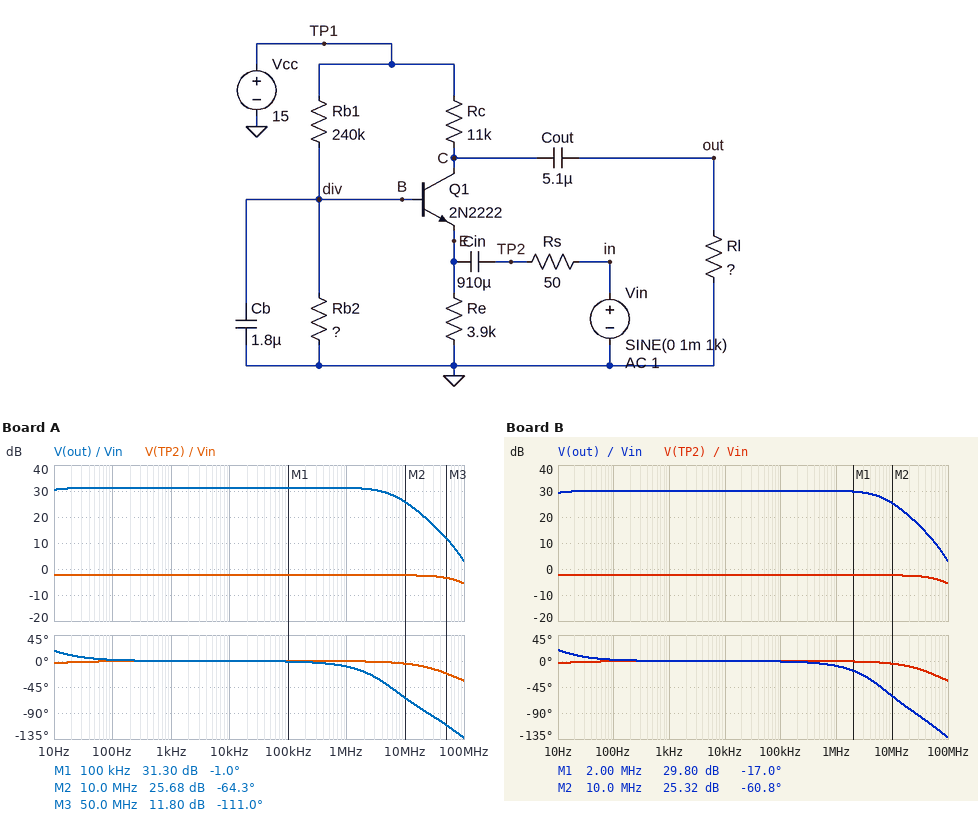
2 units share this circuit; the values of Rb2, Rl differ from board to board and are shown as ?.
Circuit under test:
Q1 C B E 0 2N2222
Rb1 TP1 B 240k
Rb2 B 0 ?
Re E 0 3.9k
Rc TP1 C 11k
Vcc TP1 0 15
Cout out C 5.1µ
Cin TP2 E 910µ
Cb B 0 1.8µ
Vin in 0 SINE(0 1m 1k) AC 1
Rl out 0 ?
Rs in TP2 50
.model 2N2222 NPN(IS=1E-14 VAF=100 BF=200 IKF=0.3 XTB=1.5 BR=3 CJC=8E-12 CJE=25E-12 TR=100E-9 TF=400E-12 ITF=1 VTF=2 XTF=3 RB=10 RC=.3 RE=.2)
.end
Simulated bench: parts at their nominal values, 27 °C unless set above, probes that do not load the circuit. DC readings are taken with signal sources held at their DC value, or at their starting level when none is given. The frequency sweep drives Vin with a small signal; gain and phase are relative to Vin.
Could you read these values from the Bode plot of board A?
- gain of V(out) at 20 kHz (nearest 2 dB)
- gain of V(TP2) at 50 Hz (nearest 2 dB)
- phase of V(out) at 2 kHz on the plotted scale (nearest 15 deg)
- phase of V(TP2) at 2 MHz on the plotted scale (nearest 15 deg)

32 dB
-2 dB
0 deg
0 deg
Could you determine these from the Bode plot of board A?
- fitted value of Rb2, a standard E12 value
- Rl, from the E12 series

22 kΩ
27 kΩ
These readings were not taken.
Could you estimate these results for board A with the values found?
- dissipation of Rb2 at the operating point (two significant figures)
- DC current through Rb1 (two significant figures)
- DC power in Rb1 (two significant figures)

70 µW
57 µA
790 µW
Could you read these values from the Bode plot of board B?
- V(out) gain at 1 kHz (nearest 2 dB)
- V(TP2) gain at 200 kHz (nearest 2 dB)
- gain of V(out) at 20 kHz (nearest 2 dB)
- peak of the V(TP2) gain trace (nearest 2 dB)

30 dB
-2 dB
30 dB
-2 dB
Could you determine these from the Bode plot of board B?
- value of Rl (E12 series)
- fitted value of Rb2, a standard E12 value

18 kΩ
22 kΩ
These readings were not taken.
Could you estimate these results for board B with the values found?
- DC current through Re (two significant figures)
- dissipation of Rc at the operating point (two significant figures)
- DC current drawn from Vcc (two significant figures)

160 µA
290 µW
220 µA
